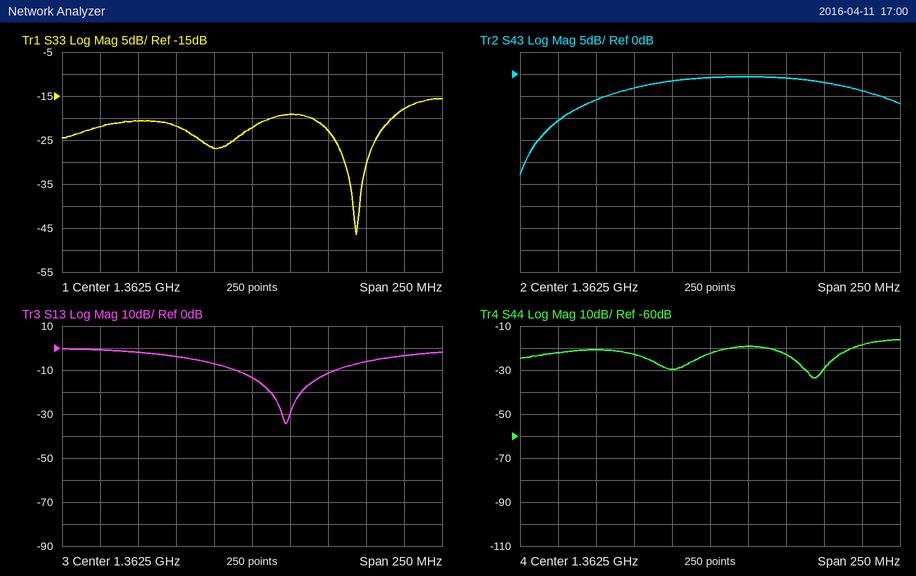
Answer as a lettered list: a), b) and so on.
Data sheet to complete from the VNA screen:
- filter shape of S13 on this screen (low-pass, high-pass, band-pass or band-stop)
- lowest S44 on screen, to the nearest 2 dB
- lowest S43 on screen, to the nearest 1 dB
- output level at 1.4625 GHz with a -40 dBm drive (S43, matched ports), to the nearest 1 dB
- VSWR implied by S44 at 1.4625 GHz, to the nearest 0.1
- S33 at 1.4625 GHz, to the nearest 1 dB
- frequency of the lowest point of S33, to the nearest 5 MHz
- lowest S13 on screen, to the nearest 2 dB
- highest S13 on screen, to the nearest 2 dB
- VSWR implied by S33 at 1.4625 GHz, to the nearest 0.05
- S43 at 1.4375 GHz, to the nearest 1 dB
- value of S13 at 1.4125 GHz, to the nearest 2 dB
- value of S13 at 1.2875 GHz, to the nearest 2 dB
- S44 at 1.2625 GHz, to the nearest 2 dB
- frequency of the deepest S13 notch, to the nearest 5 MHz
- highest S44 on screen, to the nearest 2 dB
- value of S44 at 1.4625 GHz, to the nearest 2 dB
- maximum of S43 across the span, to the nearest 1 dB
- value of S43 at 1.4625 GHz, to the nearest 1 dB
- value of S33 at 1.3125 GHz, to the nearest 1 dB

a) band-stop
b) -34 dB
c) -23 dB
d) -44 dBm
e) 1.3
f) -18 dB
g) 1.430 GHz
h) -34 dB
i) 0 dB
j) 1.30
k) -2 dB
l) -12 dB
m) -2 dB
n) -22 dB
o) 1.385 GHz
p) -16 dB
q) -18 dB
r) -1 dB
s) -4 dB
t) -22 dB
